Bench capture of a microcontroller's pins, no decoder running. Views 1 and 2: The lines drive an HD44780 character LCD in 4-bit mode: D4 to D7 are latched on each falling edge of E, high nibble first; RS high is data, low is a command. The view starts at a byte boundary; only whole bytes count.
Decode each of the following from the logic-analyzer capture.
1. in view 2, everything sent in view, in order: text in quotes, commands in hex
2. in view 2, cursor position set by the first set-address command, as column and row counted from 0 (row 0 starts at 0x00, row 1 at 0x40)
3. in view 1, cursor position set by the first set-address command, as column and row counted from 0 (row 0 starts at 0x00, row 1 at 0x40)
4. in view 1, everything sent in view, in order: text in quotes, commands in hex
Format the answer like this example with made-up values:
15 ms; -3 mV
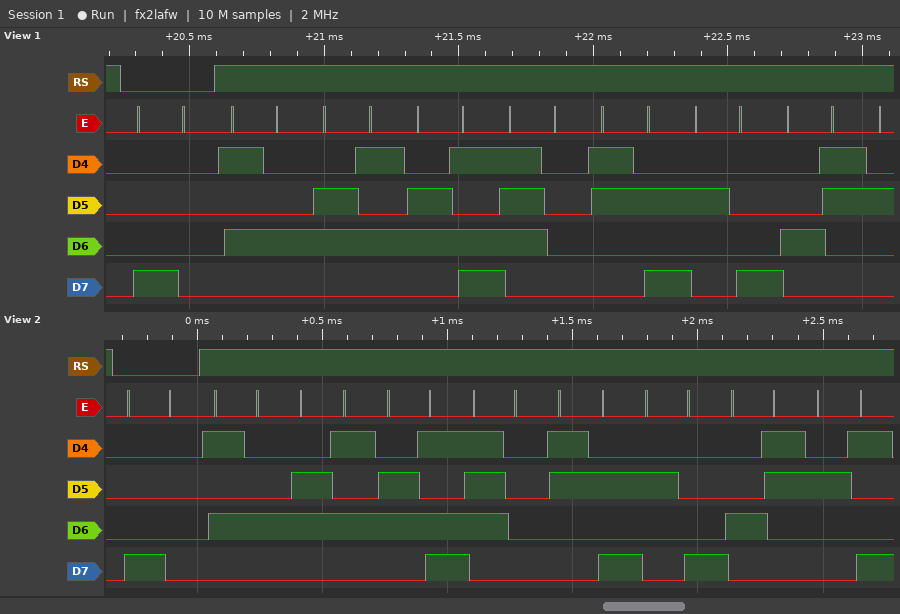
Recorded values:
0x80 "Temp:(C)"; column 0, row 0; column 0, row 0; 0x80 "Temp:(C"
